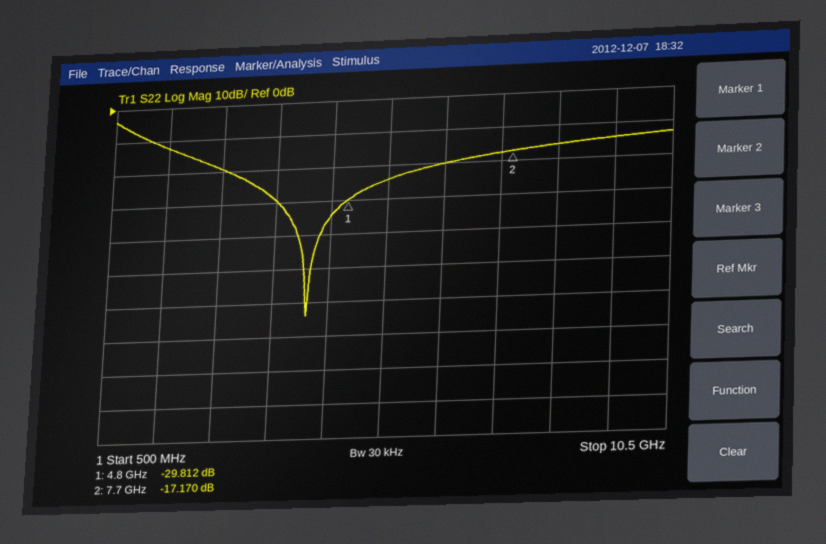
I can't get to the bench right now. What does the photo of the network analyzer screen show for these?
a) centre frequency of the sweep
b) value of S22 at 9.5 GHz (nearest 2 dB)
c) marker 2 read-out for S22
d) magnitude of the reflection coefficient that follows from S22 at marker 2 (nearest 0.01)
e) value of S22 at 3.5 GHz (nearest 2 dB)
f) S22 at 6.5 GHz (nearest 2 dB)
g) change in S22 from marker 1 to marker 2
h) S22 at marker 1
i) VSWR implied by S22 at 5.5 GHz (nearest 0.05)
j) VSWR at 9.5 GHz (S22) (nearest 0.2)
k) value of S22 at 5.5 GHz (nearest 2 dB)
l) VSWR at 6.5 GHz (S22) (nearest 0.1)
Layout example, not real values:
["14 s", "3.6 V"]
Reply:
["5.5 GHz", "-14 dB", "-17.170 dB", "0.14", "-30 dB", "-20 dB", "12.642 dB", "-29.812 dB", "1.15", "1.4", "-24 dB", "1.2"]
